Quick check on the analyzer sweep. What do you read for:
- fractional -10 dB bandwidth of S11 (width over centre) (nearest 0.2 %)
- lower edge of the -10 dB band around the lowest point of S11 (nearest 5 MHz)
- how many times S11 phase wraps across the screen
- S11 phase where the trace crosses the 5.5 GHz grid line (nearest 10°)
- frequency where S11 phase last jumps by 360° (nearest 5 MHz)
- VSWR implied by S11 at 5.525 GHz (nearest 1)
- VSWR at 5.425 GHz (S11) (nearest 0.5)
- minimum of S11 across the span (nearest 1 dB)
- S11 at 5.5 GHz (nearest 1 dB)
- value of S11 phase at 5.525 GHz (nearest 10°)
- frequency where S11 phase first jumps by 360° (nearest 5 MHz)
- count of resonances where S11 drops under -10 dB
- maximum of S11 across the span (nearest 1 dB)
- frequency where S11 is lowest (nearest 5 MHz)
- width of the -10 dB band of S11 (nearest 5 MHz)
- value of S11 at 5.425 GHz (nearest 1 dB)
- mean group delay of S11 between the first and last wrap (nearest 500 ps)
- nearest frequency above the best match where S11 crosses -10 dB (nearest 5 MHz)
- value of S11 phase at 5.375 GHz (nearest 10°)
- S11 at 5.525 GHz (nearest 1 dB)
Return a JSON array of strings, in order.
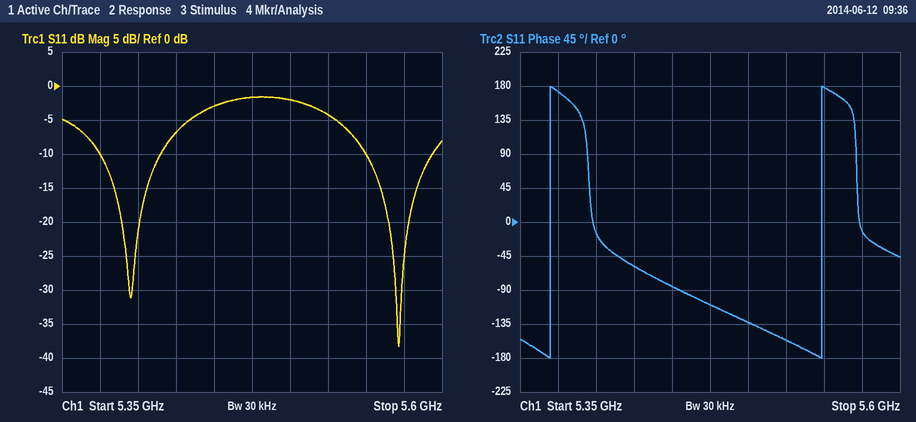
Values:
["0.8 %", "5.550 GHz", "2", "-130°", "5.550 GHz", "4", "2.5", "-38 dB", "-2 dB", "-160°", "5.370 GHz", "2", "-2 dB", "5.570 GHz", "45 MHz", "-7 dB", "5.5 ns", "5.595 GHz", "170°", "-4 dB"]
